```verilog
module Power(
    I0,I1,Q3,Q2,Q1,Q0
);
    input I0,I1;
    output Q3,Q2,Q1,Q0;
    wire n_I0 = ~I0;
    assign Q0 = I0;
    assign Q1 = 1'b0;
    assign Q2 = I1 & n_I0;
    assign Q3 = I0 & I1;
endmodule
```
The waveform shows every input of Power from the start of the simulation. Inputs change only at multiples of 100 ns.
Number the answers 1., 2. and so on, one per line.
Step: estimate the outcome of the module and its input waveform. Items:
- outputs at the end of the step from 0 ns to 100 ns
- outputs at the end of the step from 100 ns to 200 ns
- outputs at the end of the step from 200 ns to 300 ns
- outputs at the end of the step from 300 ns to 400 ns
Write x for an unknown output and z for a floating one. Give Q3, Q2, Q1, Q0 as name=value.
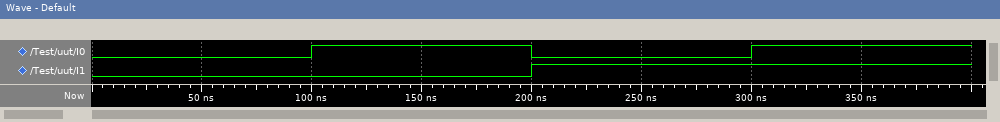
1. Q3=0, Q2=0, Q1=0, Q0=0
2. Q3=0, Q2=0, Q1=0, Q0=1
3. Q3=0, Q2=1, Q1=0, Q0=0
4. Q3=1, Q2=0, Q1=0, Q0=1
